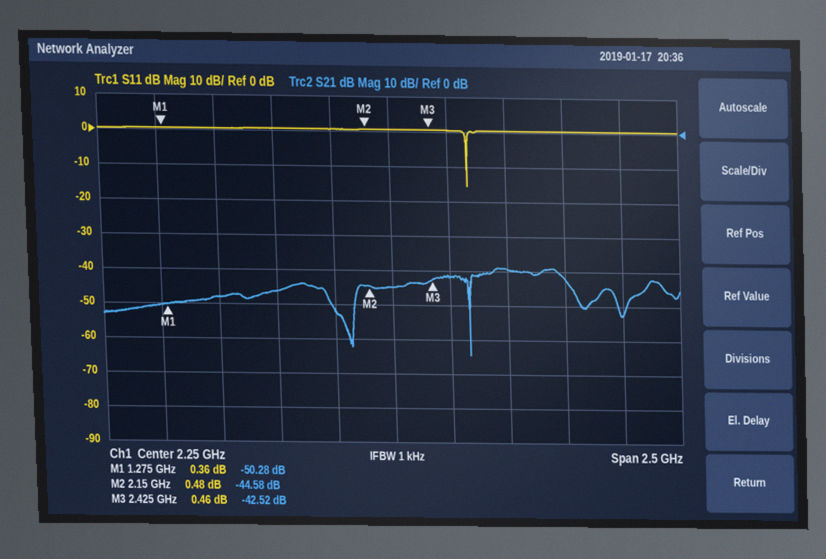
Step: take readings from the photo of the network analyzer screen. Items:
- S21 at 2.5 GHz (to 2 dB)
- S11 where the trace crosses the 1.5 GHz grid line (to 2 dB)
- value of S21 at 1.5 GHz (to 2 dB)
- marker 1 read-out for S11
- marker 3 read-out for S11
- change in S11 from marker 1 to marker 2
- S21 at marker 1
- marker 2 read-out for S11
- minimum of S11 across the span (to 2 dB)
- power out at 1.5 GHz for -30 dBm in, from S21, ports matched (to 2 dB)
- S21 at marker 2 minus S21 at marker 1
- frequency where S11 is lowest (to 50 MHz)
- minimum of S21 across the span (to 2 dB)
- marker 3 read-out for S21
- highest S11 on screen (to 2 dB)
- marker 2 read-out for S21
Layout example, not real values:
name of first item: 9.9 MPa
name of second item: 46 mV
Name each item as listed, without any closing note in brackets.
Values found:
S21 at 2.5 GHz: -42 dB
S11 where the trace crosses the 1.5 GHz grid line: 0 dB
value of S21 at 1.5 GHz: -48 dB
marker 1 read-out for S11: 0.36 dB
marker 3 read-out for S11: 0.46 dB
change in S11 from marker 1 to marker 2: 0.12 dB
S21 at marker 1: -50.28 dB
marker 2 read-out for S11: 0.48 dB
minimum of S11 across the span: -16 dB
power out at 1.5 GHz for -30 dBm in, from S21, ports matched: -78 dBm
S21 at marker 2 minus S21 at marker 1: 5.70 dB
frequency where S11 is lowest: 2.60 GHz
minimum of S21 across the span: -64 dB
marker 3 read-out for S21: -42.52 dB
highest S11 on screen: 0 dB
marker 2 read-out for S21: -44.58 dB
